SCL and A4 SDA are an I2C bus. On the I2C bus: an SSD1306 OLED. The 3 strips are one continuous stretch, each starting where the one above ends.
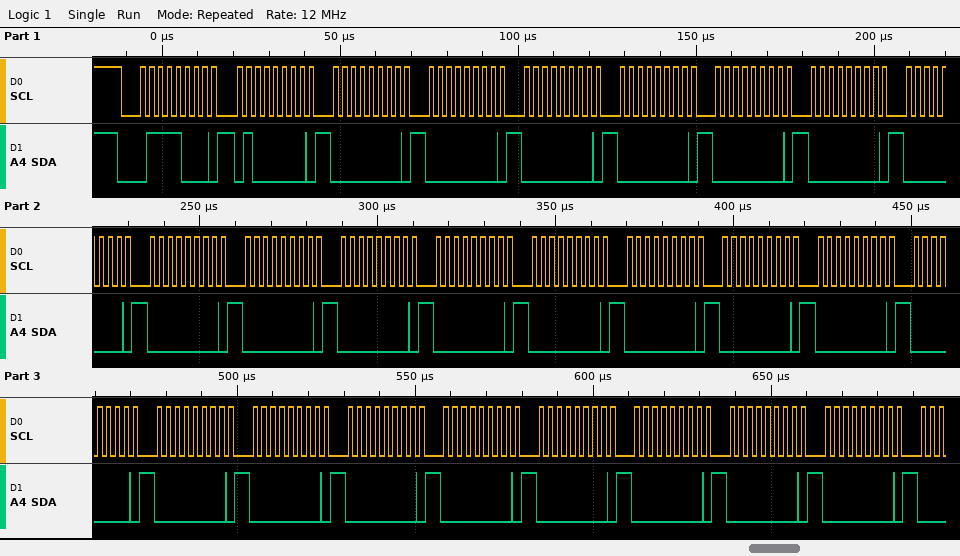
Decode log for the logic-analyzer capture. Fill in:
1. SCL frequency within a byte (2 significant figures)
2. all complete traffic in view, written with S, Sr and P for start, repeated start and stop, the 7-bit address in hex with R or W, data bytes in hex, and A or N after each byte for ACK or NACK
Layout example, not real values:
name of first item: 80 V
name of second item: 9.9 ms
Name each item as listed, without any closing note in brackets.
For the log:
SCL frequency within a byte: 400 kHz
all complete traffic in view, written with S, Sr and P for start, repeated start and stop, the 7-bit address in hex with R or W, data bytes in hex, and A or N after each byte for ACK or NACK: S 3CW A 40 A 00 A 00 A 00 A 00 A 00 A 00 A 00 A 00 A 00 A 00 A 00 A 00 A 00 A 00 A 00 A 00 A 00 A 00 A 00 A 00 A 00 A 00 A 00 A 00 A
